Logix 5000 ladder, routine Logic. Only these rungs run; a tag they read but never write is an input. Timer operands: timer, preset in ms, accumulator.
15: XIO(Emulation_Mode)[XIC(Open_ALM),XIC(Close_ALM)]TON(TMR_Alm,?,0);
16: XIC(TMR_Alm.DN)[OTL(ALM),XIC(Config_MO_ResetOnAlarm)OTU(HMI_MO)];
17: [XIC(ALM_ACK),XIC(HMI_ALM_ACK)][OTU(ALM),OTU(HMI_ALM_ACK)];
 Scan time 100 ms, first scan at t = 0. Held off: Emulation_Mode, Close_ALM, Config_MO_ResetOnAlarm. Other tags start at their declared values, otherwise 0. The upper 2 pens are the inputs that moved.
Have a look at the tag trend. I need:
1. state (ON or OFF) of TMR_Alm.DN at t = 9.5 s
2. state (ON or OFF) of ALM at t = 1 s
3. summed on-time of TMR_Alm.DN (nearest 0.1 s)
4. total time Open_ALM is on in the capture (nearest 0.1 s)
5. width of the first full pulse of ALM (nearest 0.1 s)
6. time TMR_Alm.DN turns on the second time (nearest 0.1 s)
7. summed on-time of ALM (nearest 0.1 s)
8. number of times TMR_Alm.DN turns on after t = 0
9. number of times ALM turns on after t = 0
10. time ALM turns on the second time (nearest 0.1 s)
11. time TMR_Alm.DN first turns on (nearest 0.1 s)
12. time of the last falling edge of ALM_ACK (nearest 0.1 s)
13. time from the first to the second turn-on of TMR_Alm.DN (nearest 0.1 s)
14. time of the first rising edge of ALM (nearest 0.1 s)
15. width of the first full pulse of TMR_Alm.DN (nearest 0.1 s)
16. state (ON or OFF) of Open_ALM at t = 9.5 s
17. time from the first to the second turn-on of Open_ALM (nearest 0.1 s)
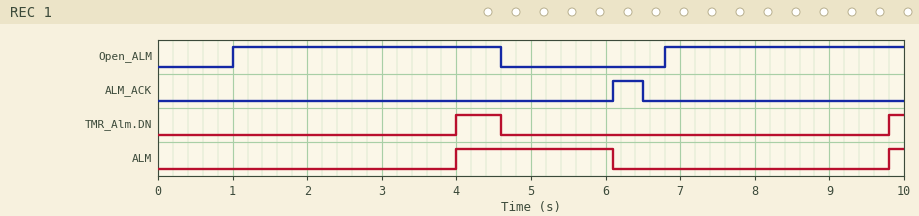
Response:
OFF
OFF
0.8 s
6.8 s
2.1 s
9.8 s
2.3 s
2
2
9.8 s
4.0 s
6.5 s
5.8 s
4.0 s
0.6 s
ON
5.8 s
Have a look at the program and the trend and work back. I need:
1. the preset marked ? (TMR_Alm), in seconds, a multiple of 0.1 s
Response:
3.0 s
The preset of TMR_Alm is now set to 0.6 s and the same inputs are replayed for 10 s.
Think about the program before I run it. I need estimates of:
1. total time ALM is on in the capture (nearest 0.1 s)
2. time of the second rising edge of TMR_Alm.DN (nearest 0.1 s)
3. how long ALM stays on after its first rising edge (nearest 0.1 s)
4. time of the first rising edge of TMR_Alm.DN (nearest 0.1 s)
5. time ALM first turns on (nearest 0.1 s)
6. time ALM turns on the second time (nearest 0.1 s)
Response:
7.1 s
7.4 s
4.5 s
1.6 s
1.6 s
7.4 s
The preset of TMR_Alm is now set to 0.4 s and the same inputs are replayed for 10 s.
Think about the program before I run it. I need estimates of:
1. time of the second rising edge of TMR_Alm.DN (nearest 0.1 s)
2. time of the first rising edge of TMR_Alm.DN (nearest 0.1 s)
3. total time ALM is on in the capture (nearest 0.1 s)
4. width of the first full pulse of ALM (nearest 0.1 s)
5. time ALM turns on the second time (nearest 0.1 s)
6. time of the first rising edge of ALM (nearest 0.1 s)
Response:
7.2 s
1.4 s
7.5 s
4.7 s
7.2 s
1.4 s
